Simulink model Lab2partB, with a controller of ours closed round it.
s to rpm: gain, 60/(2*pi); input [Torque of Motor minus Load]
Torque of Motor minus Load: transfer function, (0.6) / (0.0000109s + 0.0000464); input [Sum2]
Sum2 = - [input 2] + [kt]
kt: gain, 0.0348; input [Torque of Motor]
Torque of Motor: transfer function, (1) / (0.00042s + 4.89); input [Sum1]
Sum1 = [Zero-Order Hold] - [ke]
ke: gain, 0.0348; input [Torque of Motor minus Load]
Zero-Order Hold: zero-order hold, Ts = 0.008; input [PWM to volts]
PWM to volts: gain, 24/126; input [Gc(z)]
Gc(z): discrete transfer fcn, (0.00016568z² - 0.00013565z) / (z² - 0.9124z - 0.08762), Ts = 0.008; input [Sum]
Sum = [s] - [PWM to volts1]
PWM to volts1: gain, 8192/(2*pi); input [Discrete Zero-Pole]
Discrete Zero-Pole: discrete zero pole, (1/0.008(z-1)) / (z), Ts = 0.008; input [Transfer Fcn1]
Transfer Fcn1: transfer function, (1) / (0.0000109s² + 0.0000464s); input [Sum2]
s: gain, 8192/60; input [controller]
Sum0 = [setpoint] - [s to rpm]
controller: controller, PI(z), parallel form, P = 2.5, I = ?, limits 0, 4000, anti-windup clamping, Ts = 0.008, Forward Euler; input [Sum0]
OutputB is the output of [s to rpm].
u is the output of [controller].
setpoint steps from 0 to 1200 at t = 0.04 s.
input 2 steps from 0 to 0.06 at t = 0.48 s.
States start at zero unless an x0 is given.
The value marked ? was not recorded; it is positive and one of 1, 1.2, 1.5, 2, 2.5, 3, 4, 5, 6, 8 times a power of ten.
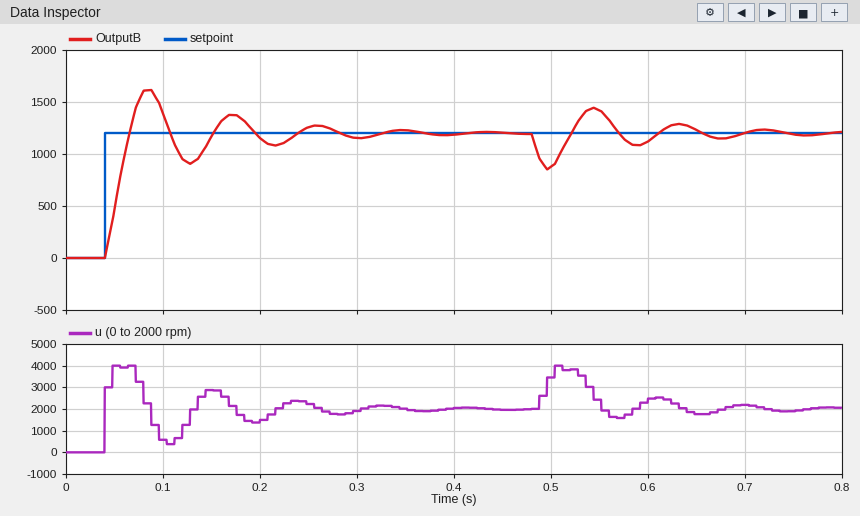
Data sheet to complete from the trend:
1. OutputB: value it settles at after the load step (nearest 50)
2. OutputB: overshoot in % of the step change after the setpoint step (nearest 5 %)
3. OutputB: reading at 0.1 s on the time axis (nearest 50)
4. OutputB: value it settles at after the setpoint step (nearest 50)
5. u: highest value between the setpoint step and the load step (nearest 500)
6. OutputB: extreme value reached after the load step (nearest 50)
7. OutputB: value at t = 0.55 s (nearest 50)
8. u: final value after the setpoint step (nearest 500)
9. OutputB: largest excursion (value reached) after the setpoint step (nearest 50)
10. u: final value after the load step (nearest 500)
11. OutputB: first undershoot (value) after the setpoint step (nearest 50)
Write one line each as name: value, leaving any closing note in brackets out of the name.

OutputB: value it settles at after the load step: 1200
OutputB: overshoot in % of the step change after the setpoint step: 35 %
OutputB: reading at 0.1 s on the time axis: 1400
OutputB: value it settles at after the setpoint step: 1200
u: highest value between the setpoint step and the load step: 4000
OutputB: extreme value reached after the load step: 850
OutputB: value at t = 0.55 s: 1400
u: final value after the setpoint step: 2000
OutputB: largest excursion (value reached) after the setpoint step: 1600
u: final value after the load step: 2000
OutputB: first undershoot (value) after the setpoint step: 900
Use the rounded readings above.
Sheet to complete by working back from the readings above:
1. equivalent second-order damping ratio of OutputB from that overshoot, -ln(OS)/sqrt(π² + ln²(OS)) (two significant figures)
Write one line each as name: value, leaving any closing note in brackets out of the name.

equivalent second-order damping ratio of OutputB from that overshoot, -ln(OS)/sqrt(π² + ln²(OS)): 0.32
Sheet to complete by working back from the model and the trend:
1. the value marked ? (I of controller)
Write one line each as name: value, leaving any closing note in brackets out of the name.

the value marked ?: 300
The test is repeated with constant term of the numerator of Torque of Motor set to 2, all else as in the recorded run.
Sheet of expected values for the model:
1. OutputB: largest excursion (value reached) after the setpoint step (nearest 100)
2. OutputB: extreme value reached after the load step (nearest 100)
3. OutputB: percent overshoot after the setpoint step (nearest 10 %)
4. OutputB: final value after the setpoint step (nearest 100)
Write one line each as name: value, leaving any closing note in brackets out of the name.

OutputB: largest excursion (value reached) after the setpoint step: 1400
OutputB: extreme value reached after the load step: 1000
OutputB: percent overshoot after the setpoint step: 20 %
OutputB: final value after the setpoint step: 1200
